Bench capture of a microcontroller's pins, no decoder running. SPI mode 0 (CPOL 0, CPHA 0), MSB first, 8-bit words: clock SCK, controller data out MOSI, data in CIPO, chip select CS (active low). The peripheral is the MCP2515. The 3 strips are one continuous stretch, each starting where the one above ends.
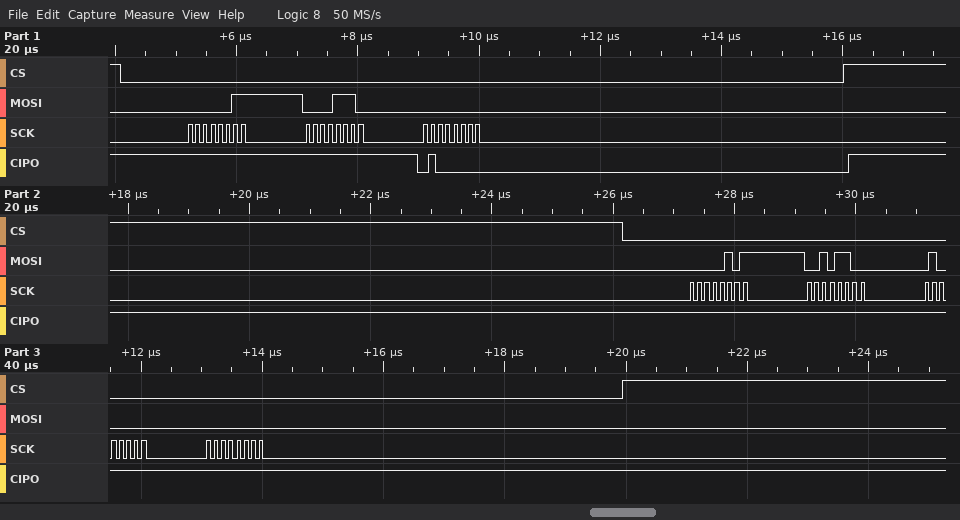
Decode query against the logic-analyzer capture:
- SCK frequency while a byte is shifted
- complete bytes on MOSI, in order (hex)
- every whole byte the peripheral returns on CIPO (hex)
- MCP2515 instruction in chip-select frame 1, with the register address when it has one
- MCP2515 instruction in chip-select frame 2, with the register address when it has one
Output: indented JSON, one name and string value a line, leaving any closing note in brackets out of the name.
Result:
{
  "SCK frequency while a byte is shifted": "8 MHz",
  "complete bytes on MOSI, in order": "03 0E 00 05 2C 40 00",
  "every whole byte the peripheral returns on CIPO": "FF FF 40 FF FF FF FF",
  "MCP2515 instruction in chip-select frame 1, with the register address when it has one": "READ 0x0E",
  "MCP2515 instruction in chip-select frame 2, with the register address when it has one": "BIT MODIFY 0x2C"
}
